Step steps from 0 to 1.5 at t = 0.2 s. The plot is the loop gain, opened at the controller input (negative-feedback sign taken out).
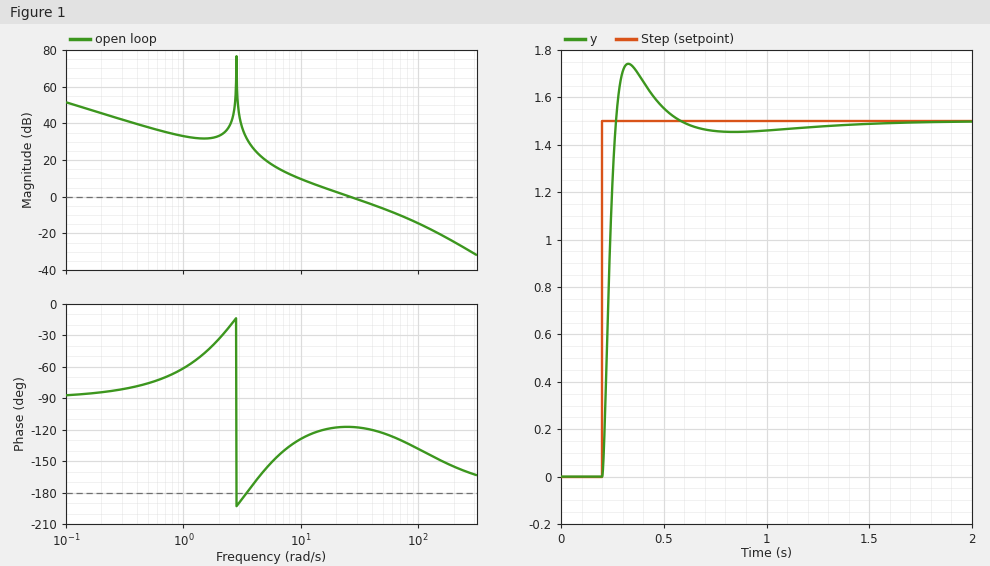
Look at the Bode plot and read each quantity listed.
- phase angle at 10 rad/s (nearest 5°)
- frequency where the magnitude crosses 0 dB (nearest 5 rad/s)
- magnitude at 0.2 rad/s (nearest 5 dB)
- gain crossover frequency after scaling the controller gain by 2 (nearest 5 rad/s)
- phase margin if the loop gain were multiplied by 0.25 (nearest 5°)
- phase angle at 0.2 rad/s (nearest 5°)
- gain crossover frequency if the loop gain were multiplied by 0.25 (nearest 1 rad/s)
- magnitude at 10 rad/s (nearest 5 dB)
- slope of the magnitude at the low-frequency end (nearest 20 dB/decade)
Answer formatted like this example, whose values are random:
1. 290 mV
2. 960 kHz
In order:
1. -130°
2. 25 rad/s
3. 45 dB
4. 50 rad/s
5. 45°
6. -85°
7. 8 rad/s
8. 10 dB
9. -20 dB/decade
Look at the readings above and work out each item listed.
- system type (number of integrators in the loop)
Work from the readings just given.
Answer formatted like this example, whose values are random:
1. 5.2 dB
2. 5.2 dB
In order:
1. 1
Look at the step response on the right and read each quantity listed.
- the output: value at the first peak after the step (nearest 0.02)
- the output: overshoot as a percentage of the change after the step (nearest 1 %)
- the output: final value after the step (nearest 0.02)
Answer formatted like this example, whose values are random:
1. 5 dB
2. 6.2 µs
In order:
1. 1.74
2. 16 %
3. 1.50
